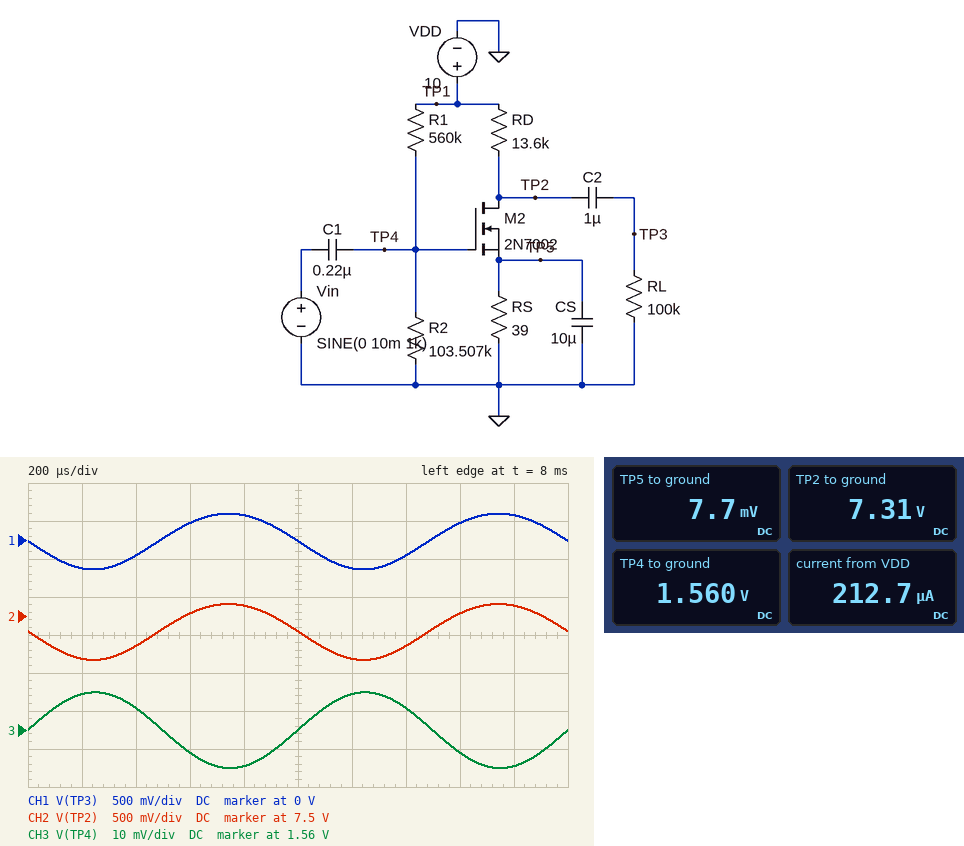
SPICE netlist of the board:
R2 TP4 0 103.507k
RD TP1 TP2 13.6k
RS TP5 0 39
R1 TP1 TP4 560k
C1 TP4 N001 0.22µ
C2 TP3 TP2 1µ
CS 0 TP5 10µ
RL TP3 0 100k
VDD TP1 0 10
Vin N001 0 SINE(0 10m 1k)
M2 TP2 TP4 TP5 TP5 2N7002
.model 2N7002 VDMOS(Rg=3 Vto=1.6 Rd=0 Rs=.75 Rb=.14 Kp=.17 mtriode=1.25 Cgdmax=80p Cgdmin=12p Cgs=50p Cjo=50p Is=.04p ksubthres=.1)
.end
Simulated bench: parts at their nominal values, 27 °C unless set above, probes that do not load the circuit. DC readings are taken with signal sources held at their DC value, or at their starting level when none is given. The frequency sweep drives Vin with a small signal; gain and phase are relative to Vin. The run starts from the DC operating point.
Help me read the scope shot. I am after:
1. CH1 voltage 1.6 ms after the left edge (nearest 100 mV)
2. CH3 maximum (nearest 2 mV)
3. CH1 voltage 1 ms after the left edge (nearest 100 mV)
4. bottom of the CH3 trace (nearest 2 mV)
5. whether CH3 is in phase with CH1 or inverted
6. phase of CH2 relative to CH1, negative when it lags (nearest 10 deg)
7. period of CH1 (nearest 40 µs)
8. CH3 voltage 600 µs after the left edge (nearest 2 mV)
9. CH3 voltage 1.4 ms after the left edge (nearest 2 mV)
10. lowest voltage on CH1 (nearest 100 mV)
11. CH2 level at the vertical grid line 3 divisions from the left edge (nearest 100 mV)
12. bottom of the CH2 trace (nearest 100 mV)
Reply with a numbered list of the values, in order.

1. 200 mV
2. 1.570 V
3. 0 V
4. 1.550 V
5. inverted
6. 0 deg
7. 1.00 ms
8. 1.554 V
9. 1.566 V
10. -400 mV
11. 7.5 V
12. 6.9 V
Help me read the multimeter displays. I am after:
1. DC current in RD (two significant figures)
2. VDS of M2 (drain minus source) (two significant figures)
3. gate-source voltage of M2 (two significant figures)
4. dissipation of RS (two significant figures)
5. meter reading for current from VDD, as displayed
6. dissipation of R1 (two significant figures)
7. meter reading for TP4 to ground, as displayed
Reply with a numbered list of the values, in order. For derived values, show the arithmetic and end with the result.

1. (10 V - 7.31 V) / 13.6 kΩ = 200 µA
2. 7.31 V - 7.7 mV = 7.3 V
3. 1.56 V - 7.7 mV = 1.6 V
4. (7.7 mV)^2 / 39 Ω = 1.5 µW
5. 212.7 µA
6. (10 V - 1.56 V)^2 / 560 kΩ = 130 µW
7. 1.560 V
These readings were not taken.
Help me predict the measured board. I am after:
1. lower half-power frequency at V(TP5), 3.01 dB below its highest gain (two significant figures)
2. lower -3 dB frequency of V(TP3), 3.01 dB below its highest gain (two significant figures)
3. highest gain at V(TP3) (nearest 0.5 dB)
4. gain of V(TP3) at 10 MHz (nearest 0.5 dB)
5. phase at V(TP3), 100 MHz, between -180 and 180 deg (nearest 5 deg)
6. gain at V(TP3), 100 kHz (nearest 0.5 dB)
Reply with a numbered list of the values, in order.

1. 8.0 Hz
2. 11 Hz
3. 31.5 dB
4. 4.0 dB
5. 10 deg
6. 31.0 dB
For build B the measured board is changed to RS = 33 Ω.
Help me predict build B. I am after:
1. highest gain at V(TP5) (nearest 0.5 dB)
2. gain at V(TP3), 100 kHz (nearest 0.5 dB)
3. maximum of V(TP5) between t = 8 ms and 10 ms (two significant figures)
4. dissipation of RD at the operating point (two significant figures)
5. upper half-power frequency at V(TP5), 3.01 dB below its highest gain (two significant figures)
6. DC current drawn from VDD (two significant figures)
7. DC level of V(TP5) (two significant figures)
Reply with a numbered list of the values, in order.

1. -20.5 dB
2. 31.5 dB
3. 7.1 mV
4. 550 µW
5. 550 Hz
6. 220 µA
7. 6.6 mV
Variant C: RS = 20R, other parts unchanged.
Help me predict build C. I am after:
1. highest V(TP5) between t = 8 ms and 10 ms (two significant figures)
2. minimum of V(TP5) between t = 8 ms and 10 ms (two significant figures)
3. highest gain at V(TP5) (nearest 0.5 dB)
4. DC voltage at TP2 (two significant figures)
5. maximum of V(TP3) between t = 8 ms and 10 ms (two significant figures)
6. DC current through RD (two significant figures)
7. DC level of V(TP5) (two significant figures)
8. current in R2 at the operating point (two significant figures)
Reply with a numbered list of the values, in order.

1. 4.6 mV
2. 3.8 mV
3. -24.5 dB
4. 7.2 V
5. 360 mV
6. 210 µA
7. 4.2 mV
8. 15 µA
